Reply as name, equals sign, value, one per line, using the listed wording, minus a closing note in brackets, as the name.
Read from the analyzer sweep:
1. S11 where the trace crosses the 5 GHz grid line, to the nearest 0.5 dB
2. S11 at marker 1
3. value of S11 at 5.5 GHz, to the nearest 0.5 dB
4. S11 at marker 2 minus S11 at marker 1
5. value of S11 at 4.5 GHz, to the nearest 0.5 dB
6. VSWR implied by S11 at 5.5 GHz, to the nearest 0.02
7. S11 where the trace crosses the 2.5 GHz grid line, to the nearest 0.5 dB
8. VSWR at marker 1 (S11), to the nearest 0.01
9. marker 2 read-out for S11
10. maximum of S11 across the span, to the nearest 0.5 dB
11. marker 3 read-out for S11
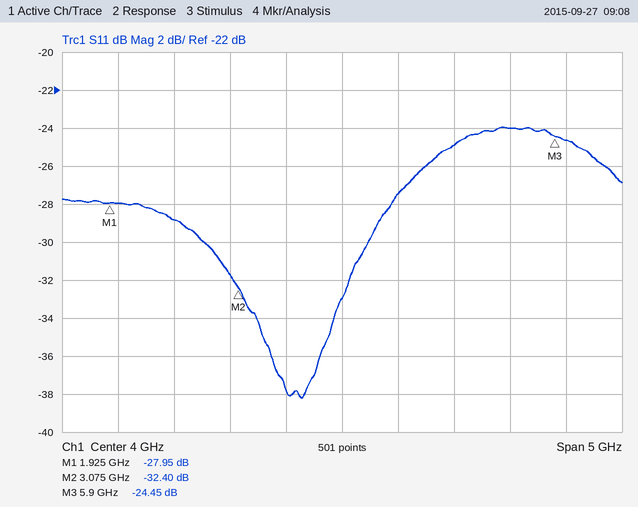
S11 where the trace crosses the 5 GHz grid line, to the nearest 0.5 dB = -25.0 dB
S11 at marker 1 = -27.95 dB
value of S11 at 5.5 GHz, to the nearest 0.5 dB = -24.0 dB
S11 at marker 2 minus S11 at marker 1 = -4.45 dB
value of S11 at 4.5 GHz, to the nearest 0.5 dB = -27.5 dB
VSWR implied by S11 at 5.5 GHz, to the nearest 0.02 = 1.14
S11 where the trace crosses the 2.5 GHz grid line, to the nearest 0.5 dB = -29.0 dB
VSWR at marker 1 (S11), to the nearest 0.01 = 1.08
marker 2 read-out for S11 = -32.40 dB
maximum of S11 across the span, to the nearest 0.5 dB = -24.0 dB
marker 3 read-out for S11 = -24.45 dB
